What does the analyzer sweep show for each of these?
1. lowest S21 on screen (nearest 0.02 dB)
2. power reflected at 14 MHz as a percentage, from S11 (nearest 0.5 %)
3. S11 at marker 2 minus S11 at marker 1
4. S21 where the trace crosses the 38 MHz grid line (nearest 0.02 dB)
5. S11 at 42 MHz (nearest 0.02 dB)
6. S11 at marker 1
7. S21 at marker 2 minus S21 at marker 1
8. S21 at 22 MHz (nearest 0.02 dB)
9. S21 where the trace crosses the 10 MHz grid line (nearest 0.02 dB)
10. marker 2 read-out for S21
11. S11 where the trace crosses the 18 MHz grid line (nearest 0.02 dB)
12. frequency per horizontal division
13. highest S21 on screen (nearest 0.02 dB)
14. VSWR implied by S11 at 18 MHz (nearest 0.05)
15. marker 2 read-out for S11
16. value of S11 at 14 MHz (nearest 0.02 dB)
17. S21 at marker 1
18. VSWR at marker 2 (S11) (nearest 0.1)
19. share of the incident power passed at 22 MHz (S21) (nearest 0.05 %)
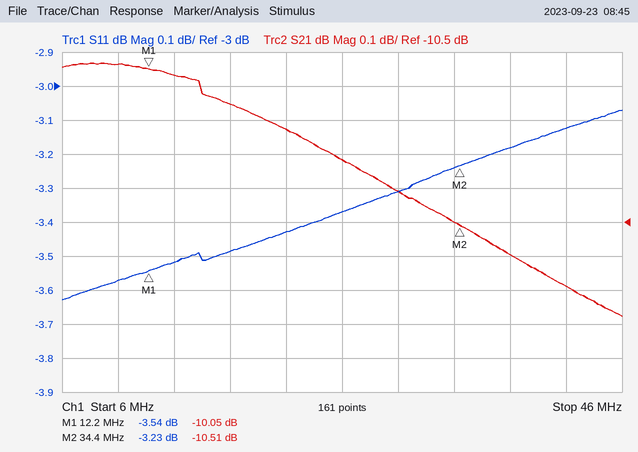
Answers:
-10.78 dB
44.5 %
0.31 dB
-10.60 dB
-3.12 dB
-3.54 dB
-0.46 dB
-10.22 dB
-10.04 dB
-10.51 dB
-3.48 dB
4 MHz
-10.04 dB
5.05
-3.23 dB
-3.52 dB
-10.05 dB
5.4
9.50 %
